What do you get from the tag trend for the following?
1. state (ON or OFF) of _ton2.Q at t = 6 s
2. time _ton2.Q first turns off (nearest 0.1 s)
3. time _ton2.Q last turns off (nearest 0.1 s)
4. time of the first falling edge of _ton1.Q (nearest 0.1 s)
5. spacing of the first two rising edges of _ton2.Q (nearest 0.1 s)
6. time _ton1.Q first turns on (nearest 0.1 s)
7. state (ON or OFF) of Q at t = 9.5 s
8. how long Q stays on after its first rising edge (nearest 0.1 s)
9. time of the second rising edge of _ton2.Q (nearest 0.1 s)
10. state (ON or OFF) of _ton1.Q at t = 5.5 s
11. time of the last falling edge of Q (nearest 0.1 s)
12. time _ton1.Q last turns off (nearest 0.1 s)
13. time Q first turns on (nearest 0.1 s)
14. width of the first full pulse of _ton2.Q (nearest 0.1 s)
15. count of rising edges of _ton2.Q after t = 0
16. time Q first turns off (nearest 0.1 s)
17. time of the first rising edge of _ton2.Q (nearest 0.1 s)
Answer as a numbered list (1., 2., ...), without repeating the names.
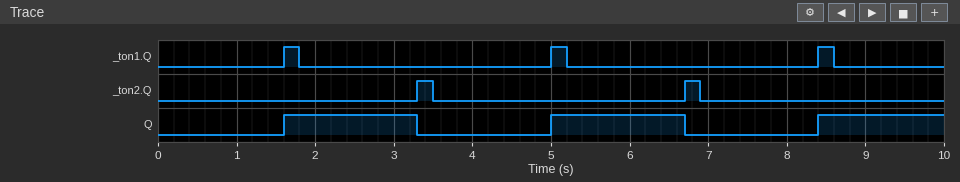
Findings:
1. OFF
2. 3.5 s
3. 6.9 s
4. 1.8 s
5. 3.4 s
6. 1.6 s
7. ON
8. 1.7 s
9. 6.7 s
10. OFF
11. 6.7 s
12. 8.6 s
13. 1.6 s
14. 0.2 s
15. 2
16. 3.3 s
17. 3.3 s
